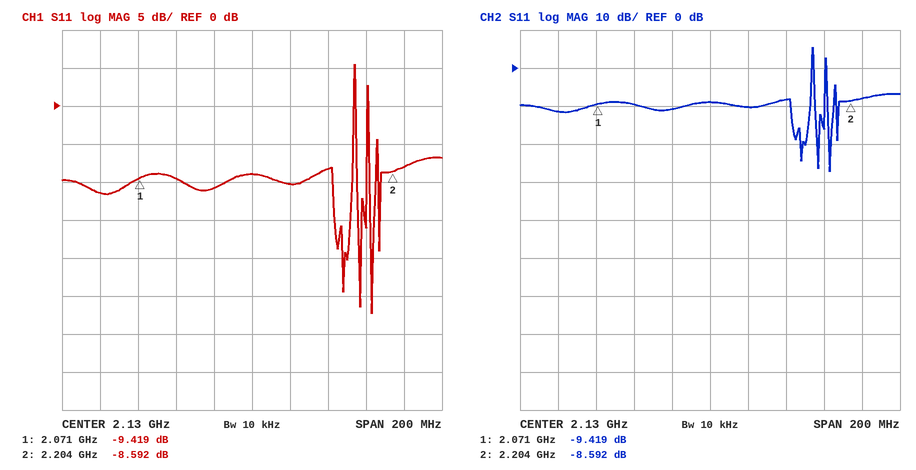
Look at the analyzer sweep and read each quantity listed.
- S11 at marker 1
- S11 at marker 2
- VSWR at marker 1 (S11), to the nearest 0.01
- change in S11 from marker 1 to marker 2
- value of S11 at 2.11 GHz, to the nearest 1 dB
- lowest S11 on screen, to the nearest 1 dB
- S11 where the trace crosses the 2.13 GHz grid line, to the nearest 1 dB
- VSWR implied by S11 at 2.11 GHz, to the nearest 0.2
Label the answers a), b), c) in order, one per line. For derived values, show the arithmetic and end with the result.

a) -9.419 dB
b) -8.592 dB
c) (1 + 0.3381)/(1 − 0.3381) ≈ 2.02
d) -8.592 − (-9.419) = 0.827 dB
e) -11 dB
f) -27 dB
g) -9 dB
h) |Γ| = 10^(-11/20) = 0.2818; VSWR = (1 + 0.2818)/(1 − 0.2818) ≈ 1.8
